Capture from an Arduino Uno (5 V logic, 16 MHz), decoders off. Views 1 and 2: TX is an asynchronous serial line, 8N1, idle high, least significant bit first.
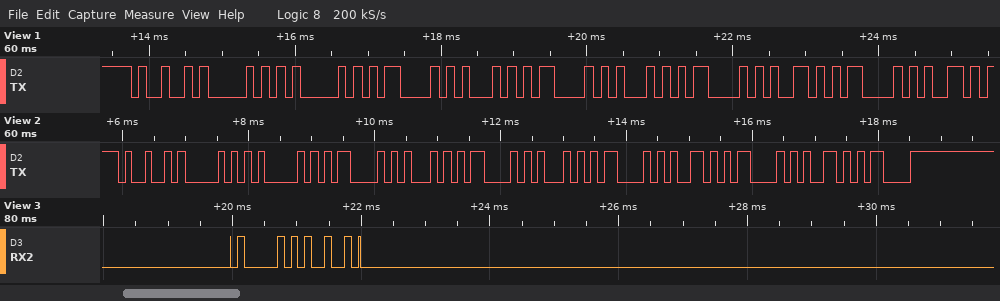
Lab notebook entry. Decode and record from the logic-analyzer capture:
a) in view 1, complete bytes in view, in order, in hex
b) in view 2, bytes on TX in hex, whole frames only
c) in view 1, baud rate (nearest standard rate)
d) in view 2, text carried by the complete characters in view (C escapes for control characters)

49 50 41 0D 45 0D 45 0D 65 0D 65
0x49 0x50 0x41 0x0D 0x45 0x0D 0x45 0x0D 0x65 0x0D 0x65 0x0D
9600 baud
"IPA\rE\rE\re\re\r"
